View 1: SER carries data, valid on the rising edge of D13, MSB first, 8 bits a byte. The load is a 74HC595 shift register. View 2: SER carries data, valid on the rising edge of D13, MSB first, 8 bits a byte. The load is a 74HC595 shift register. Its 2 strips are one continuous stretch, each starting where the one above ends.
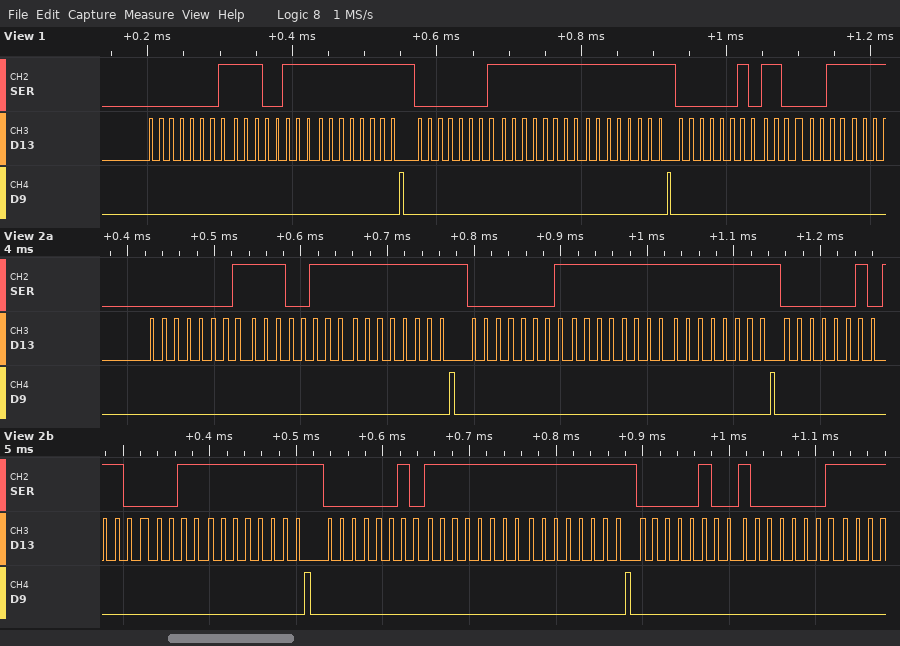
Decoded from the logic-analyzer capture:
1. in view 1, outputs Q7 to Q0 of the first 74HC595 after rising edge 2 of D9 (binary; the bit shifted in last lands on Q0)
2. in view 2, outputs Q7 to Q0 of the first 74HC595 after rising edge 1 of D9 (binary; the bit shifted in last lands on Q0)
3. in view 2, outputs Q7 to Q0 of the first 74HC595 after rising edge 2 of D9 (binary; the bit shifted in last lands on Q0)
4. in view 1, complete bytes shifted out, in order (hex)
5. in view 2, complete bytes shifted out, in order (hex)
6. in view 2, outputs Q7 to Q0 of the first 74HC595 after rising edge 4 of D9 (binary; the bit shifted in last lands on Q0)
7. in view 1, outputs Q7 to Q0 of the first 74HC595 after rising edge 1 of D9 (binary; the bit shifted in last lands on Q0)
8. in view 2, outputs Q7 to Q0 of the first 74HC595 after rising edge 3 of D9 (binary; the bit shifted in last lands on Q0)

11111111
11111111
11111111
01 E7 FF 01 FF FF 02 C3
0x01 0xE7 0xFF 0x01 0xFF 0xFF 0x02 0xC3 0xFF 0x02 0xFF 0xFF 0x04 0x81
11111111
11111111
11111111
